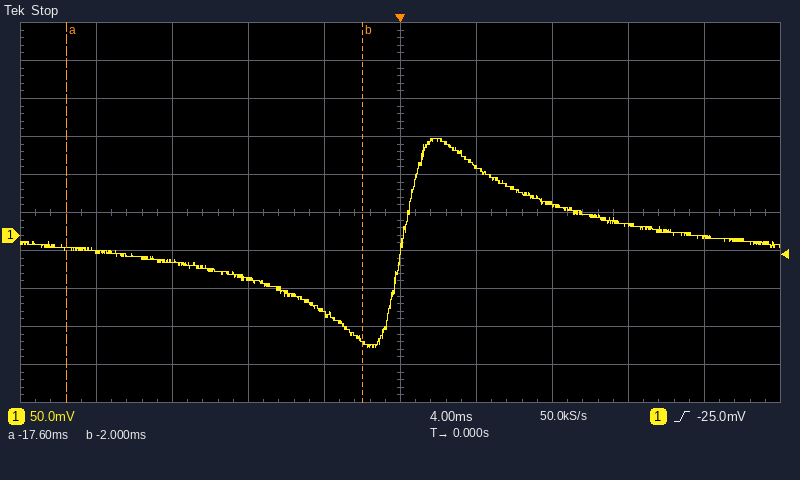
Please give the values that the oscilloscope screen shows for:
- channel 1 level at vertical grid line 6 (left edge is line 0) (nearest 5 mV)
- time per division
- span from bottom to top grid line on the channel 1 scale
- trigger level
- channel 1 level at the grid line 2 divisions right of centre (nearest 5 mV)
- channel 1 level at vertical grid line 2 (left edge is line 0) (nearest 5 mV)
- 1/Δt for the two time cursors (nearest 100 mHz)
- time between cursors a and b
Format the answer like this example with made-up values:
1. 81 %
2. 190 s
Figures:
1. 90 mV
2. 4 ms
3. 500 mV
4. -25.0 mV
5. 40 mV
6. -35 mV
7. 64.1 Hz
8. 15.6 ms
